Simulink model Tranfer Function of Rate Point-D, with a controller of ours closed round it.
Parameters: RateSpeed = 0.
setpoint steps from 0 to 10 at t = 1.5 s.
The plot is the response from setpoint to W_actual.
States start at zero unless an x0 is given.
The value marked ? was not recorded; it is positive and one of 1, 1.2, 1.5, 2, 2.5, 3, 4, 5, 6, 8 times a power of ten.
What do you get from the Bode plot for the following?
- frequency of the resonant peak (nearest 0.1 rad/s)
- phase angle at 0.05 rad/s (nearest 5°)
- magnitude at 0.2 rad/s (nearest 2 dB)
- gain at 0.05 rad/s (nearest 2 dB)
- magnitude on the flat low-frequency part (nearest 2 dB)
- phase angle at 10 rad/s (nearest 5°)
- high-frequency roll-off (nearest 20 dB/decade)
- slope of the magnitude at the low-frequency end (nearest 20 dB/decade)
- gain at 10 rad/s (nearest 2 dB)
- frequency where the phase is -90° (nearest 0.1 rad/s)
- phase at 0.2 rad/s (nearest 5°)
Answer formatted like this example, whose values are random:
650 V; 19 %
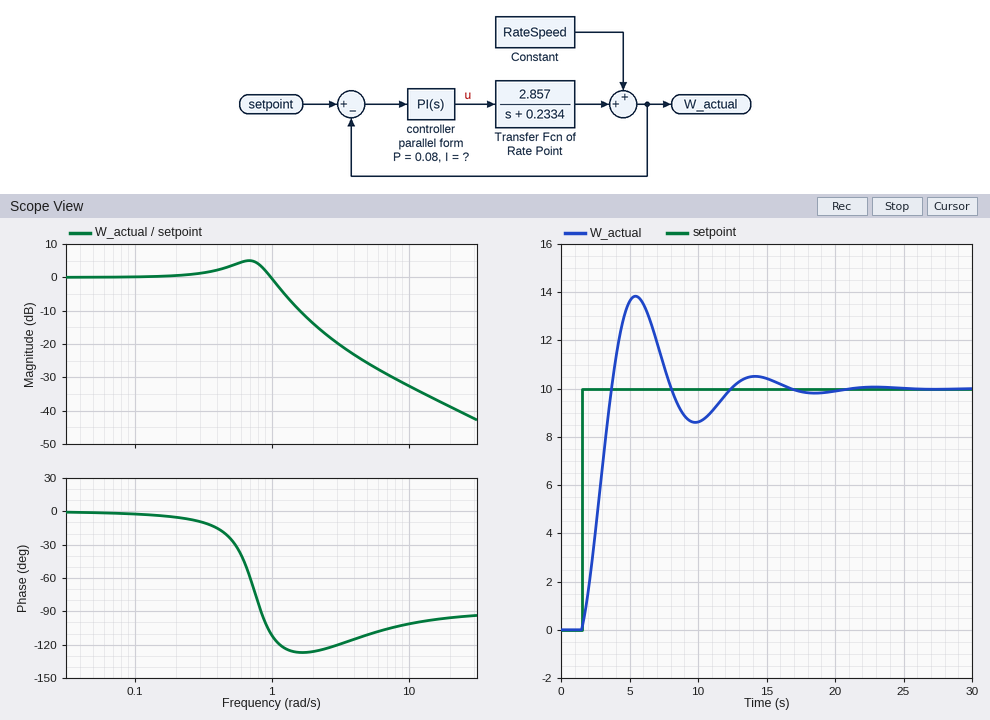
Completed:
0.7 rad/s; 0°; 0 dB; 0 dB; 0 dB; -100°; -20 dB/decade; 0 dB/decade; -32 dB; 0.8 rad/s; -5°
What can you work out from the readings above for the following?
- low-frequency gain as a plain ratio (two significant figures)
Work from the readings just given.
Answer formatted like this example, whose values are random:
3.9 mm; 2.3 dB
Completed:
1.0
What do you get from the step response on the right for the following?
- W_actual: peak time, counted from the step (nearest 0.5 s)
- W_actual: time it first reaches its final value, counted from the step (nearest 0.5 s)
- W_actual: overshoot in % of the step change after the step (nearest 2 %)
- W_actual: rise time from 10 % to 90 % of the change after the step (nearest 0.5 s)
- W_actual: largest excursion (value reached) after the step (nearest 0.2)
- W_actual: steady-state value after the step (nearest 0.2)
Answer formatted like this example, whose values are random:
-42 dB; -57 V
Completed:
4.0 s; 2.0 s; 38 %; 1.5 s; 13.8; 10.0
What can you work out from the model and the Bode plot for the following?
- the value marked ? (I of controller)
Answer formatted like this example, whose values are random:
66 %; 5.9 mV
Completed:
0.2
